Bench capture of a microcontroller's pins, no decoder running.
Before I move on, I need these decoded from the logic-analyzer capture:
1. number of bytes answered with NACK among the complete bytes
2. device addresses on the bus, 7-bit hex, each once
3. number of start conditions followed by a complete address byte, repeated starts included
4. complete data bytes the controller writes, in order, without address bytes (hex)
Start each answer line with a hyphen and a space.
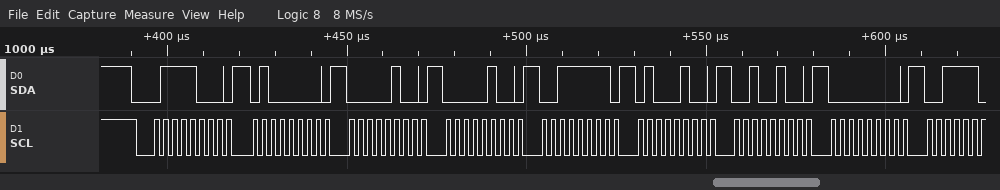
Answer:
- 0
- 0x3C
- 1
- 40 04 04 3F 44 24 00
